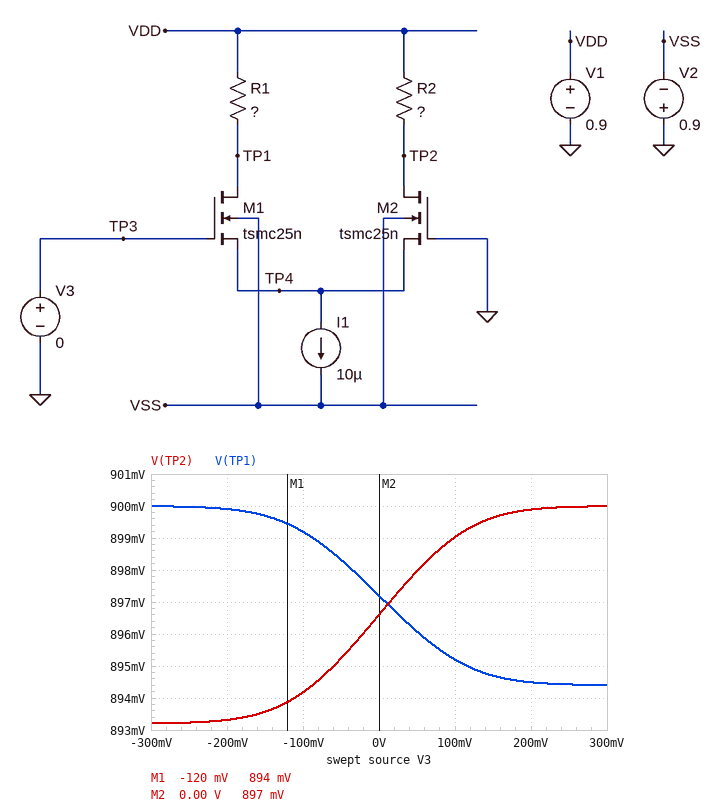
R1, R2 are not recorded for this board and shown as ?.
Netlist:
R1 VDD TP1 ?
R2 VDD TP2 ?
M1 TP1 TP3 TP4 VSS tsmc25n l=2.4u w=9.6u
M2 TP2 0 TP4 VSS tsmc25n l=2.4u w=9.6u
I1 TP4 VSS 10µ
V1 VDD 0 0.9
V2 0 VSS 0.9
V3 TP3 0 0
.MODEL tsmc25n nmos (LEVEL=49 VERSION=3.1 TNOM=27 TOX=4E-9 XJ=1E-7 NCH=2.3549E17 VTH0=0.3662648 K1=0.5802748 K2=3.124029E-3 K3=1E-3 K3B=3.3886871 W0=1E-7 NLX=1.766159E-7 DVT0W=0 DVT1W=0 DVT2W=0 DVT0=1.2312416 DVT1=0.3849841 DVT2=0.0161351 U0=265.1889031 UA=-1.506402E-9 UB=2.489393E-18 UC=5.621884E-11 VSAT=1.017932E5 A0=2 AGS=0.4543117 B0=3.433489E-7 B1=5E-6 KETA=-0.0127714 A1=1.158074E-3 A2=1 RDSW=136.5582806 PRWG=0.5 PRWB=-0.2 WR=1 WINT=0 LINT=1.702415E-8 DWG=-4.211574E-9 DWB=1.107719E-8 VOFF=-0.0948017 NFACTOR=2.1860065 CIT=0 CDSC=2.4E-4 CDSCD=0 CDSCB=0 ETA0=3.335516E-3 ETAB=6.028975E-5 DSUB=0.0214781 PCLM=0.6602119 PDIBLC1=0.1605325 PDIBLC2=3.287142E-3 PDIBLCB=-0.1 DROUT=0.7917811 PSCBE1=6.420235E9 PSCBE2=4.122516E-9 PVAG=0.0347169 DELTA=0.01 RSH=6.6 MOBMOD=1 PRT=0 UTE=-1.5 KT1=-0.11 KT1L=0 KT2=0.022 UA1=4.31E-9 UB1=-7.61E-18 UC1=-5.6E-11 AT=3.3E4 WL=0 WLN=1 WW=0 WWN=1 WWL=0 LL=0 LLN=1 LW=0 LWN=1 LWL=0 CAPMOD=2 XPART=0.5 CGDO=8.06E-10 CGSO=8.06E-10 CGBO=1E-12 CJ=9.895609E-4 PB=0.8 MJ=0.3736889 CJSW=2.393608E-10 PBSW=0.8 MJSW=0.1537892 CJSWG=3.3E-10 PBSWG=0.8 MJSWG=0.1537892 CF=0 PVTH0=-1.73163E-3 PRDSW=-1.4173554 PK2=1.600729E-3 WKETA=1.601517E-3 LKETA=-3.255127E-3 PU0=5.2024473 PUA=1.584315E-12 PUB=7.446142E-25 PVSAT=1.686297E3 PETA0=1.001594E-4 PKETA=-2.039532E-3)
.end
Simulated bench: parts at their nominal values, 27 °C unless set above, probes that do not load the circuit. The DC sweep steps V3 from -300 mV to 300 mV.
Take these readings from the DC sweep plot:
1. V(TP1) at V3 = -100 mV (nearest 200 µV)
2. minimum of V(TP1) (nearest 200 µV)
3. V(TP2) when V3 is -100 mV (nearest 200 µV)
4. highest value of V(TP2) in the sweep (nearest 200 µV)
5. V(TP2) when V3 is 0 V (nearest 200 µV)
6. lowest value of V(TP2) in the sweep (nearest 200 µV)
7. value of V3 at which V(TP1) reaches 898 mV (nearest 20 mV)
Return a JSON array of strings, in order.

["899.2 mV", "894.4 mV", "894.2 mV", "900.0 mV", "896.6 mV", "893.2 mV", "-40 mV"]
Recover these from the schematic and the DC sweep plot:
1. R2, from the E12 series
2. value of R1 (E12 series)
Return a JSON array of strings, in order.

["680 Ω", "560 Ω"]
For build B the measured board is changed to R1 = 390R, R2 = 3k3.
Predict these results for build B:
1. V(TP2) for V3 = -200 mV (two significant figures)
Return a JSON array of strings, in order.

["870 mV"]
